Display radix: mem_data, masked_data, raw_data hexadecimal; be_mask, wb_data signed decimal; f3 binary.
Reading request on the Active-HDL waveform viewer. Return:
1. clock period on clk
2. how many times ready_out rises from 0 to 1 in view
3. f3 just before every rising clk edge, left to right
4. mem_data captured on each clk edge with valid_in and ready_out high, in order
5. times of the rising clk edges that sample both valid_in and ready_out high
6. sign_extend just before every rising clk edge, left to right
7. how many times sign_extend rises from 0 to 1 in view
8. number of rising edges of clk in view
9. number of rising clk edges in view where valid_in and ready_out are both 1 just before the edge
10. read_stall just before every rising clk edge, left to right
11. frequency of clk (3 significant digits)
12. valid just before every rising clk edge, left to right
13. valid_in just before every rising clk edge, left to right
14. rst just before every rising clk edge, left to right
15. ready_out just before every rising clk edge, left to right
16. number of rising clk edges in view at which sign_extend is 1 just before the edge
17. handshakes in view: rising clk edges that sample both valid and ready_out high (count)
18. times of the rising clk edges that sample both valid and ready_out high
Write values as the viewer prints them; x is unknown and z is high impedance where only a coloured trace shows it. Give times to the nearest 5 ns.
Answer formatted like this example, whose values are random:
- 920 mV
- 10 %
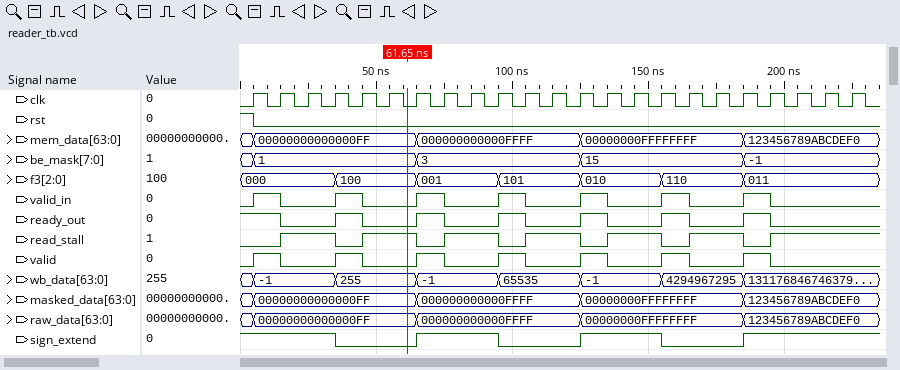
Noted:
- 10 ns
- 6
- 000, 000, 000, 000, 100, 100, 100, 001, 001, 001, 101, 101, 101, 010, 010, 010, 110, 110, 110, 011, 011, 011, 011
- 00000000000000FF, 00000000000000FF, 000000000000FFFF, 000000000000FFFF, 00000000FFFFFFFF, 00000000FFFFFFFF, 123456789ABCDEF0
- 15 ns, 45 ns, 75 ns, 105 ns, 135 ns, 165 ns, 195 ns
- 1 1 1 1 0 0 0 1 1 1 0 0 0 1 1 1 0 0 0 1 1 1 1
- 3
- 23
- 7
- 0 0 1 1 0 1 1 0 1 1 0 1 1 0 1 1 0 1 1 0 1 1 1
- 100 MHz
- 0 1 0 0 1 0 0 1 0 0 1 0 0 1 0 0 1 0 0 1 0 0 0
- 0 1 0 0 1 0 0 1 0 0 1 0 0 1 0 0 1 0 0 1 0 0 0
- 1 0 0 0 0 0 0 0 0 0 0 0 0 0 0 0 0 0 0 0 0 0 0
- 1 1 0 0 1 0 0 1 0 0 1 0 0 1 0 0 1 0 0 1 0 0 0
- 14
- 7
- 15 ns, 45 ns, 75 ns, 105 ns, 135 ns, 165 ns, 195 ns
